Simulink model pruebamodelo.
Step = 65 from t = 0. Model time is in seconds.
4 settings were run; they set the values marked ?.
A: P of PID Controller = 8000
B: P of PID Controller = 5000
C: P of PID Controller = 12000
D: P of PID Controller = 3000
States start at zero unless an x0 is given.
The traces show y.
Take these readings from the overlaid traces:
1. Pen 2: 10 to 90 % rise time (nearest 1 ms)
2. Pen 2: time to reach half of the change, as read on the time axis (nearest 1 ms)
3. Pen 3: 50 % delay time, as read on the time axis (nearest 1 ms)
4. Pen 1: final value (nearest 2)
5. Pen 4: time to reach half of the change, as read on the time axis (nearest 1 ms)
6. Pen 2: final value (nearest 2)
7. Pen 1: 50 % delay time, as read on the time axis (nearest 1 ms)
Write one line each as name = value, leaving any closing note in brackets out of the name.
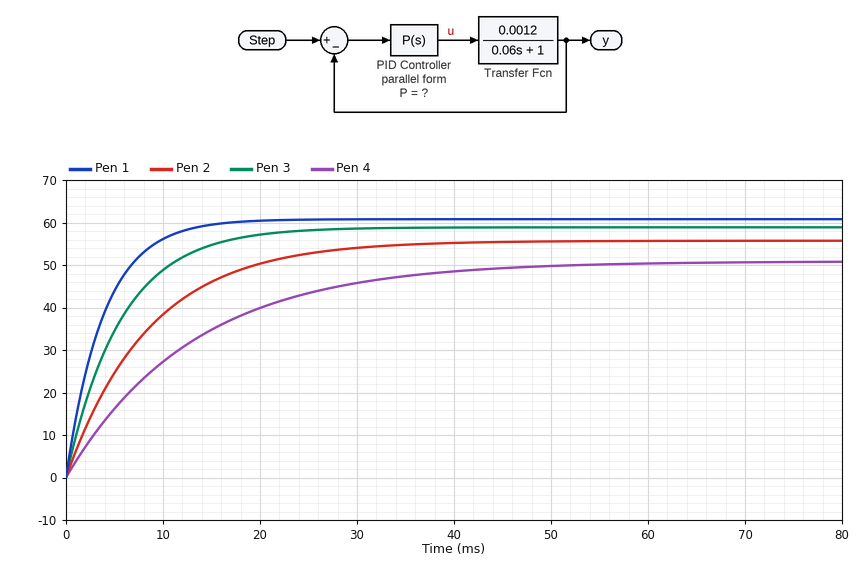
Pen 2: 10 to 90 % rise time = 19 ms
Pen 2: time to reach half of the change, as read on the time axis = 6 ms
Pen 3: 50 % delay time, as read on the time axis = 4 ms
Pen 1: final value = 60
Pen 4: time to reach half of the change, as read on the time axis = 9 ms
Pen 2: final value = 56
Pen 1: 50 % delay time, as read on the time axis = 3 ms
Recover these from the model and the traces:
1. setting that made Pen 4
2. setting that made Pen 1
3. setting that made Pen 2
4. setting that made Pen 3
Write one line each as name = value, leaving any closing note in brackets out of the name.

setting that made Pen 4 = D
setting that made Pen 1 = C
setting that made Pen 2 = B
setting that made Pen 3 = A
